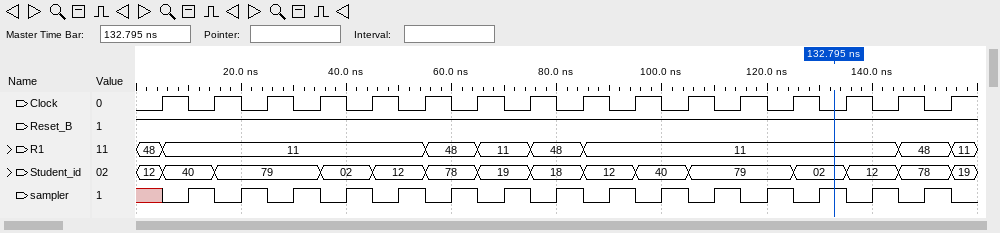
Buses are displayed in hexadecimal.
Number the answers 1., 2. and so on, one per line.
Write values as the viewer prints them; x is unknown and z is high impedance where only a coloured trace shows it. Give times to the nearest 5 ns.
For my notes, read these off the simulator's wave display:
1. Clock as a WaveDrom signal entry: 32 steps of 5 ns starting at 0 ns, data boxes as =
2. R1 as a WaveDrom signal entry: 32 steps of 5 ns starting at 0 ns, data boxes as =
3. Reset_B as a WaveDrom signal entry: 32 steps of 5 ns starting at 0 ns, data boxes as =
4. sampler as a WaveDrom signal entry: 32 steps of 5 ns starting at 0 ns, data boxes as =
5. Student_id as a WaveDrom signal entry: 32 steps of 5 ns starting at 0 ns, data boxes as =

1. {name: 'Clock', wave: '01010101010101010101010101010101'}
2. {name: 'R1', wave: '==.........=.=.=.=...........=.=', data: '48 11 48 11 48 11 48 11'}
3. {name: 'Reset_B', wave: '1...............................'}
4. {name: 'sampler', wave: 'x0101010101010101010101010101010'}
5. {name: 'Student_id', wave: '==.=...=.=.=.=.=.=.=.=...=.=.=.=', data: '12 40 79 02 12 78 19 18 12 40 79 02 12 78 19'}
